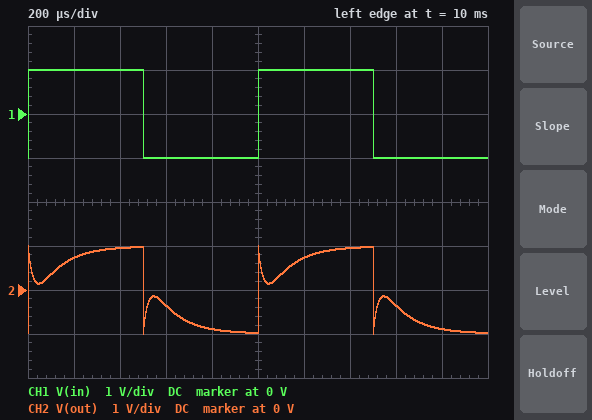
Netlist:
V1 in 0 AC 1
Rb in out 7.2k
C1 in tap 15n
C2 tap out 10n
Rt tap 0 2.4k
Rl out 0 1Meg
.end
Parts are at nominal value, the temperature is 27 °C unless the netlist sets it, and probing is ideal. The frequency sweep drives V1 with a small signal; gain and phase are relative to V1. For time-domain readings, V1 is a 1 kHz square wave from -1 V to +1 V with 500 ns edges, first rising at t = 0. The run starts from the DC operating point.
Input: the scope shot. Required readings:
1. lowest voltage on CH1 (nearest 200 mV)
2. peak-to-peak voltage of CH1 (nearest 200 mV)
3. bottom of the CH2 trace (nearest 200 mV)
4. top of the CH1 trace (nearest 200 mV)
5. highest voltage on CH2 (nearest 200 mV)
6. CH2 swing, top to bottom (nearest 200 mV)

-1.0 V
2.0 V
-1.0 V
1.0 V
1.0 V
2.0 V
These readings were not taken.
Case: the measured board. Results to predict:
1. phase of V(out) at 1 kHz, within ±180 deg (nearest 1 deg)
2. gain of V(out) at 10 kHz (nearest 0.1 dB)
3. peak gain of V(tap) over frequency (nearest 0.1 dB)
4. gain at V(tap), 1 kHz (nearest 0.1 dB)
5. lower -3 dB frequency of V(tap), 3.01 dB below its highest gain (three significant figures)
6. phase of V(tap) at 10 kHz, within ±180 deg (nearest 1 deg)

-20 deg
-1.9 dB
0 dB
-9.9 dB
4.82 kHz
22 deg
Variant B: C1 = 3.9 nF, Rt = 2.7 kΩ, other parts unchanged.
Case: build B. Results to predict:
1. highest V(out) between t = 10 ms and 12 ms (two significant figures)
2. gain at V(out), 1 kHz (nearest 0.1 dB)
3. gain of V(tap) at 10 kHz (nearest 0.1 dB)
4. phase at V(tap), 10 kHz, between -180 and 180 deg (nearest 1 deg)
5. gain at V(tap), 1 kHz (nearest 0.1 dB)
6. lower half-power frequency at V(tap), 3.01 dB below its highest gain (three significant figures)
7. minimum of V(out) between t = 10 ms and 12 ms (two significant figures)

980 mV
-1.6 dB
-5.5 dB
36 deg
-14.0 dB
18.5 kHz
-980 mV
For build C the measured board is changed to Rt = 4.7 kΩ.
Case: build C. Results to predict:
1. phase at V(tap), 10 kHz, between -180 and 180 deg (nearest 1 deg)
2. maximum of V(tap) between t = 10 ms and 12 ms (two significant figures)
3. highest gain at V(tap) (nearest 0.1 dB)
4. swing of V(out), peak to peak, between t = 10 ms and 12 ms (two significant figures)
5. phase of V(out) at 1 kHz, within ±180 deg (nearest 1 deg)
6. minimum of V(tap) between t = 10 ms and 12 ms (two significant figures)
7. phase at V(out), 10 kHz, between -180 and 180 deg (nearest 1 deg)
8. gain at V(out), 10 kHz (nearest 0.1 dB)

12 deg
1.9 V
0 dB
2.1 V
-13 deg
-1.9 V
11 deg
-0.8 dB
